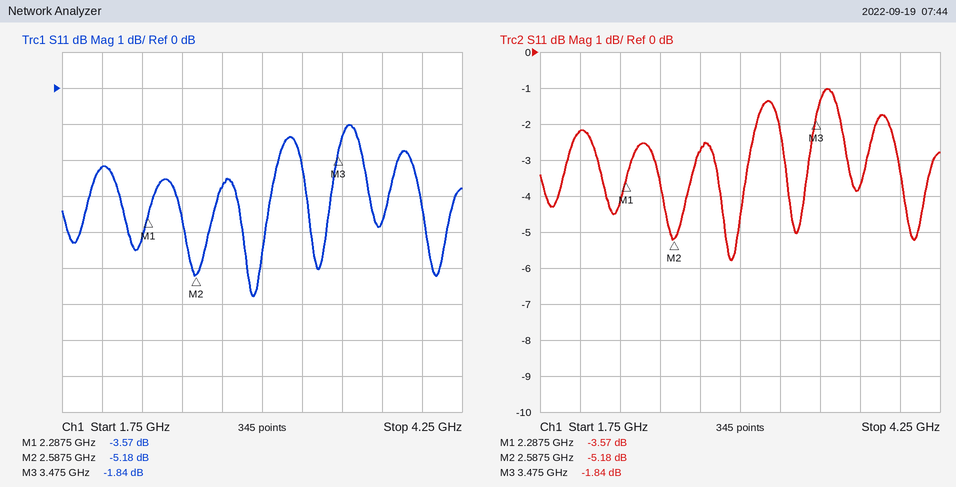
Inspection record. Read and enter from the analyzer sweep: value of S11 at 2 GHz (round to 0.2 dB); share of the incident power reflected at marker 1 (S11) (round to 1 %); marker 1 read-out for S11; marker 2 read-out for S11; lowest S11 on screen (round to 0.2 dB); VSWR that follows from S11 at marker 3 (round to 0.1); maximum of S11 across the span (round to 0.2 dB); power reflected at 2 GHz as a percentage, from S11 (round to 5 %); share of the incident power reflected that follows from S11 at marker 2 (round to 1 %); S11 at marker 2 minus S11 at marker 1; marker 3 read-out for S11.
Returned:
-2.2 dB
44 %
-3.57 dB
-5.18 dB
-5.8 dB
9.5
-1.0 dB
60 %
30 %
-1.61 dB
-1.84 dB
